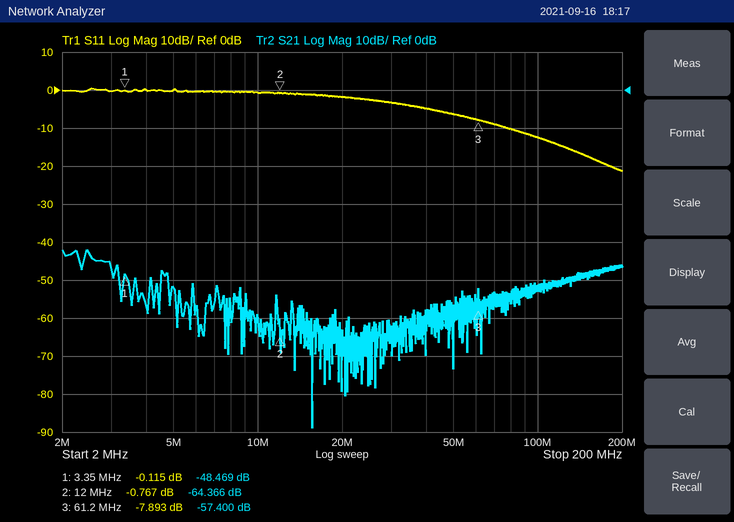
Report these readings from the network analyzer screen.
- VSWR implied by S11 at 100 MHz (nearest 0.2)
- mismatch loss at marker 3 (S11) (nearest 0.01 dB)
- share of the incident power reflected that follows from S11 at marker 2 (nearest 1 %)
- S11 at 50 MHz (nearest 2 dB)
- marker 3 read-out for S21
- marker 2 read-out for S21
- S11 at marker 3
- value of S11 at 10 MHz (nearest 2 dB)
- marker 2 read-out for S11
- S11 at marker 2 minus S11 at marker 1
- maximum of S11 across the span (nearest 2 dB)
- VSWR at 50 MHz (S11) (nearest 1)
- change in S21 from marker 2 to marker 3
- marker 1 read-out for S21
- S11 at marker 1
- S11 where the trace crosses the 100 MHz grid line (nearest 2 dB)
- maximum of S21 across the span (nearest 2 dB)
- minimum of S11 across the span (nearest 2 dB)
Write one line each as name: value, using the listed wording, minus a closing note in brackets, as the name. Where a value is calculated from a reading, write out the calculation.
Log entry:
VSWR implied by S11 at 100 MHz: |Γ| = 10^(-12/20) = 0.2512; VSWR = (1 + 0.2512)/(1 − 0.2512) ≈ 1.67, so 1.6 to the nearest 0.2
mismatch loss at marker 3 (S11): −10 log10(1 − 10^(-7.893/10)) ≈ 0.77 dB
share of the incident power reflected that follows from S11 at marker 2: 10^(-0.767/10) ≈ 84 %
S11 at 50 MHz: -6 dB
marker 3 read-out for S21: -57.400 dB
marker 2 read-out for S21: -64.366 dB
S11 at marker 3: -7.893 dB
value of S11 at 10 MHz: 0 dB
marker 2 read-out for S11: -0.767 dB
S11 at marker 2 minus S11 at marker 1: -0.767 − (-0.115) = -0.652 dB
maximum of S11 across the span: 0 dB
VSWR at 50 MHz (S11): |Γ| = 10^(-6/20) = 0.5012; VSWR = (1 + 0.5012)/(1 − 0.5012) ≈ 3
change in S21 from marker 2 to marker 3: -57.4 − (-64.366) = 6.966 dB
marker 1 read-out for S21: -48.469 dB
S11 at marker 1: -0.115 dB
S11 where the trace crosses the 100 MHz grid line: -12 dB
maximum of S21 across the span: -42 dB
minimum of S11 across the span: -22 dB
